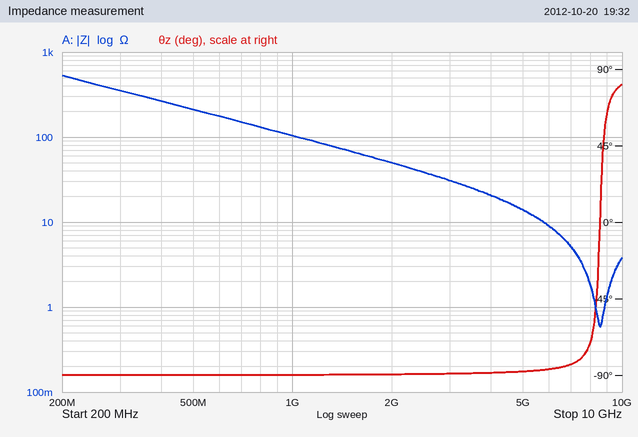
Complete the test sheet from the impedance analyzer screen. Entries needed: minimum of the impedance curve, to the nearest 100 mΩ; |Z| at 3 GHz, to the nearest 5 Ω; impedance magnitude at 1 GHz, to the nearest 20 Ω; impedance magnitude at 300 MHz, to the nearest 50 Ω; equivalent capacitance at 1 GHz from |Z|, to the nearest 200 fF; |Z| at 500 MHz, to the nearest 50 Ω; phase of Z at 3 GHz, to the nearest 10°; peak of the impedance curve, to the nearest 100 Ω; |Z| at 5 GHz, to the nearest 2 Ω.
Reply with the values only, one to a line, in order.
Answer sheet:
600 mΩ
30 Ω
100 Ω
350 Ω
1.6 pF
200 Ω
-90°
500 Ω
14 Ω
